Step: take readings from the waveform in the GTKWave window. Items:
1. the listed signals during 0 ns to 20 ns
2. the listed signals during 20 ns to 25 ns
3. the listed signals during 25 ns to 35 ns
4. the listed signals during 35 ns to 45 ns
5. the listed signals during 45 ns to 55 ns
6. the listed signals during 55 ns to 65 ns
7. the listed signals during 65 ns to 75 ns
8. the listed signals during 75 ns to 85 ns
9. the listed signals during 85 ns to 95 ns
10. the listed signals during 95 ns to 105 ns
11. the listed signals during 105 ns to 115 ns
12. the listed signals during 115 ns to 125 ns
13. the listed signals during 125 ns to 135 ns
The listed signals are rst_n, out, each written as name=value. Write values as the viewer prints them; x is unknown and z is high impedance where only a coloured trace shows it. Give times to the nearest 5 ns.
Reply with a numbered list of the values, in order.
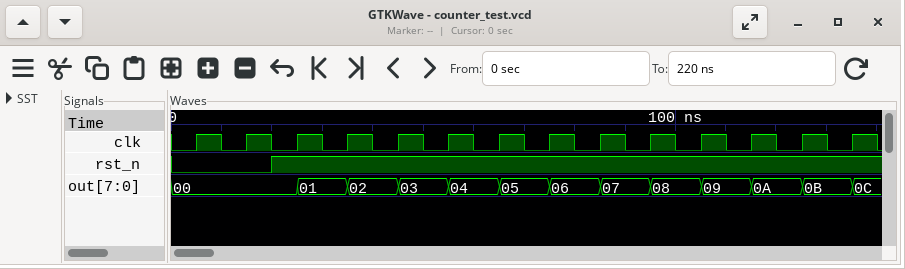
1. rst_n=0, out=00
2. rst_n=1, out=00
3. rst_n=1, out=01
4. rst_n=1, out=02
5. rst_n=1, out=03
6. rst_n=1, out=04
7. rst_n=1, out=05
8. rst_n=1, out=06
9. rst_n=1, out=07
10. rst_n=1, out=08
11. rst_n=1, out=09
12. rst_n=1, out=0A
13. rst_n=1, out=0B
